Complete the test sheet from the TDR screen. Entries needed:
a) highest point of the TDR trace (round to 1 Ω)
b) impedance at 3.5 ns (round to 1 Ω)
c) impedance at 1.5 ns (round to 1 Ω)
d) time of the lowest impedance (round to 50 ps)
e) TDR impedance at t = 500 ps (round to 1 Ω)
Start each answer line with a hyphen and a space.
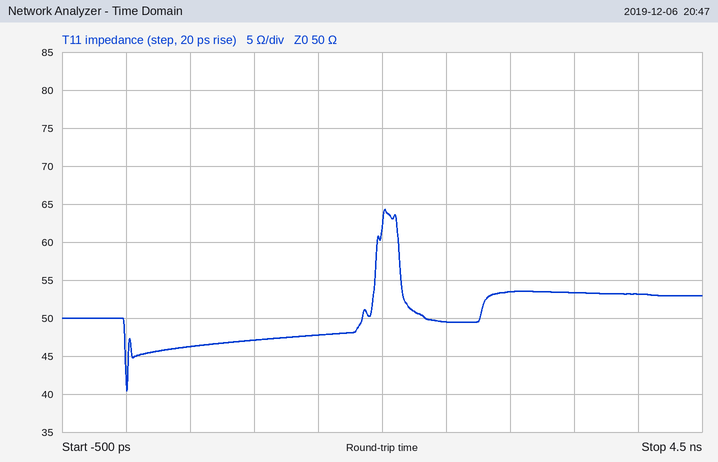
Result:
- 64 Ω
- 53 Ω
- 48 Ω
- 0 ps
- 46 Ω
